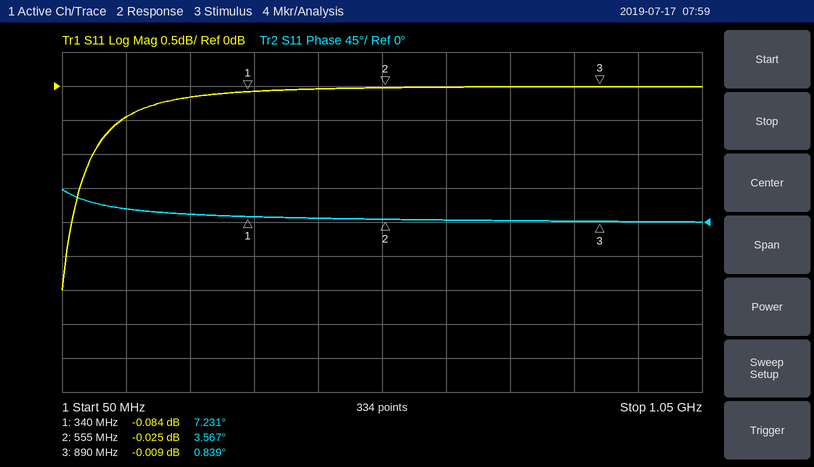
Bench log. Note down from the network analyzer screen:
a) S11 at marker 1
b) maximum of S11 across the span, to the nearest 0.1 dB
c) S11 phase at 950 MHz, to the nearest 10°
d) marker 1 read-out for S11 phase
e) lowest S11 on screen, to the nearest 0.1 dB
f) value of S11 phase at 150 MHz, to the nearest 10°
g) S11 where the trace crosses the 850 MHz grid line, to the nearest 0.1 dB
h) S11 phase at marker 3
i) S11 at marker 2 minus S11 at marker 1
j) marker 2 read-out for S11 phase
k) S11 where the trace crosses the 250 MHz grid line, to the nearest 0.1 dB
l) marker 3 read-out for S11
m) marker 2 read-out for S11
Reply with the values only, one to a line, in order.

-0.084 dB
0.0 dB
0°
7.231°
-3.0 dB
20°
0.0 dB
0.839°
0.059 dB
3.567°
-0.2 dB
-0.009 dB
-0.025 dB
